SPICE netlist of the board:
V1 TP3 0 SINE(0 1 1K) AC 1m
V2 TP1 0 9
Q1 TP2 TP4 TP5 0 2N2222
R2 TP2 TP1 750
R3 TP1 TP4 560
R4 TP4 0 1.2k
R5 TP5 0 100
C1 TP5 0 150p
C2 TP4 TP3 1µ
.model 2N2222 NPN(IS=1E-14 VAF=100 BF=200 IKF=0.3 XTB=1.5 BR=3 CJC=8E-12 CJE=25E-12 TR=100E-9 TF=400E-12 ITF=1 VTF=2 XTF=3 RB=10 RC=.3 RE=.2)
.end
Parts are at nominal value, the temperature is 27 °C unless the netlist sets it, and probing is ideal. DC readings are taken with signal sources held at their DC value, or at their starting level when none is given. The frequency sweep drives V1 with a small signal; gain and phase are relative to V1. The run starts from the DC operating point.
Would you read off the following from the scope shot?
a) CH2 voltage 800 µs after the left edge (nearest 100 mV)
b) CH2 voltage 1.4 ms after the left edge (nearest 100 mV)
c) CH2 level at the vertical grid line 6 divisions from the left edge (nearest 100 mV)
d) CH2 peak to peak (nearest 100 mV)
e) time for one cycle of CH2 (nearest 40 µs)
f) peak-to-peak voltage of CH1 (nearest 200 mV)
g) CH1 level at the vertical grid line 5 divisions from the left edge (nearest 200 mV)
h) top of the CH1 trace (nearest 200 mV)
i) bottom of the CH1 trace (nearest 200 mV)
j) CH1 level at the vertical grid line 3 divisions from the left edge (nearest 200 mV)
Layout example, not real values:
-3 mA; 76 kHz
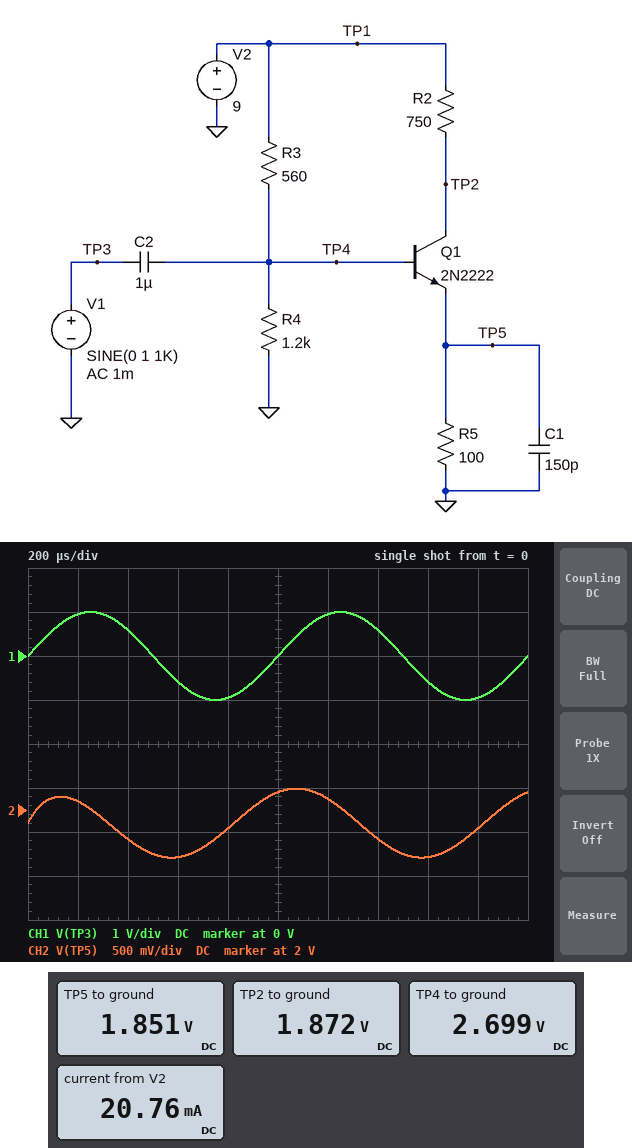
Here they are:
1.8 V; 1.7 V; 2.1 V; 800 mV; 1.00 ms; 2.0 V; 0 V; 1.0 V; -1.0 V; -600 mV
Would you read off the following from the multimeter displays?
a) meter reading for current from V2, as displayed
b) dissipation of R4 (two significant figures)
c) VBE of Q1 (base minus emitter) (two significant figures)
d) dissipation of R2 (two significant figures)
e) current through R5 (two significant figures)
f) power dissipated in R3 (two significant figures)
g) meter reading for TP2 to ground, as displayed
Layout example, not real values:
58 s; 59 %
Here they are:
20.76 mA; 6.1 mW; 850 mV; 68 mW; 19 mA; 71 mW; 1.872 V
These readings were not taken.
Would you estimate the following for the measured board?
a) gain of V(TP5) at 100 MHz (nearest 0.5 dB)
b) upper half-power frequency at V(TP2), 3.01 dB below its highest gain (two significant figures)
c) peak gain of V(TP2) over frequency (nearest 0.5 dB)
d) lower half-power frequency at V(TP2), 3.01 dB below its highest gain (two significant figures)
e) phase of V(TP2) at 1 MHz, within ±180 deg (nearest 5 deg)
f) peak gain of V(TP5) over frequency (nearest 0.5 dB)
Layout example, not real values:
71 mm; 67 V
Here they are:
-3.5 dB; 110 MHz; -1.0 dB; 2.1 kHz; 0 deg; -1.0 dB
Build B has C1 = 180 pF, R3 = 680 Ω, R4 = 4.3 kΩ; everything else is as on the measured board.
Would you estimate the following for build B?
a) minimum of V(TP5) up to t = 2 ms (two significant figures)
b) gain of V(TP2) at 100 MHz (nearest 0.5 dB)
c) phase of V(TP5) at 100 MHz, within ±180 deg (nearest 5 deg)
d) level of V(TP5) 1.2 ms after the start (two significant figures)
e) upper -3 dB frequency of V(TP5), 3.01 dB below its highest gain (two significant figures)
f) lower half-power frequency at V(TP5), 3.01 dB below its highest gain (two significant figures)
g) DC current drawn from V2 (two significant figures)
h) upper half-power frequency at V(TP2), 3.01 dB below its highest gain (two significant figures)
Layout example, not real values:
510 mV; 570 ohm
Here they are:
1.4 V; -4.0 dB; -45 deg; 2.1 V; 91 MHz; 1.9 kHz; 19 mA; 94 MHz
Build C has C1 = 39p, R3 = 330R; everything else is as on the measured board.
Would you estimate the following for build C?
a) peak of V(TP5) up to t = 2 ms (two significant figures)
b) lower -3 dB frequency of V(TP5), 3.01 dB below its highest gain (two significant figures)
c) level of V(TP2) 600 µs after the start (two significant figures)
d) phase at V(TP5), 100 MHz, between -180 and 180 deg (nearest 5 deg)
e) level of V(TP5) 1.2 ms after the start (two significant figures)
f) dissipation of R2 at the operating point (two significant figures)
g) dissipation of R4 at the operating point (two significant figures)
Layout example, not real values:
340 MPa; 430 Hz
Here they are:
2.7 V; 2.3 kHz; 2.0 V; -15 deg; 2.6 V; 59 mW; 8.9 mW
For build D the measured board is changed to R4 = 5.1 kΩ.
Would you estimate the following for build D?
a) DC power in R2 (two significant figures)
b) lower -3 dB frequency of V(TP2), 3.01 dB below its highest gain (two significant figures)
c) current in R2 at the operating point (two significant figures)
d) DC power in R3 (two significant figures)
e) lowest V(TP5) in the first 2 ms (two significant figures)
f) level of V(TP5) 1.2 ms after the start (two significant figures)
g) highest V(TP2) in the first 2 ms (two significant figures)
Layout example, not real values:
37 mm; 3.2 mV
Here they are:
65 mW; 2.0 kHz; 9.3 mA; 68 mW; 1.6 V; 2.3 V; 2.4 V
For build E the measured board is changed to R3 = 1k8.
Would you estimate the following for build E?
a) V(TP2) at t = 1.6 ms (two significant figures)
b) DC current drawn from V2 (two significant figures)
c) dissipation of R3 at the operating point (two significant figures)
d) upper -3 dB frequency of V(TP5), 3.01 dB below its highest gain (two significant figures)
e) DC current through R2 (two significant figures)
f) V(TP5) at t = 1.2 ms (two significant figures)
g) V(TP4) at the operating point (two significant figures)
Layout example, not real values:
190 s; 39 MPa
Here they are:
5.2 V; 14 mA; 27 mW; 100 MHz; 10 mA; 1.6 V; 2.0 V
